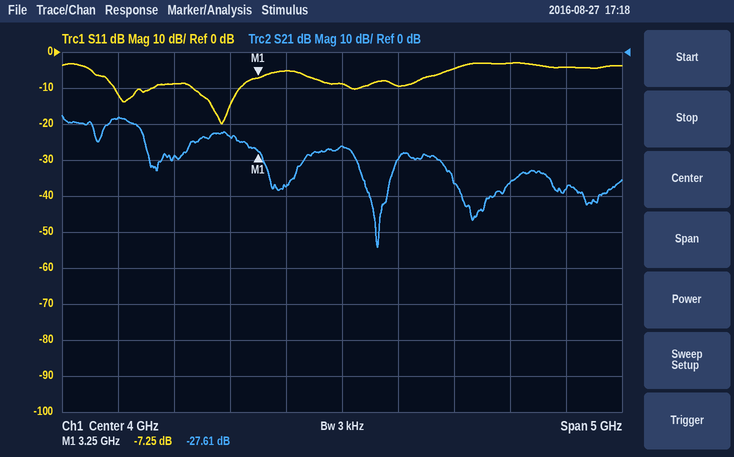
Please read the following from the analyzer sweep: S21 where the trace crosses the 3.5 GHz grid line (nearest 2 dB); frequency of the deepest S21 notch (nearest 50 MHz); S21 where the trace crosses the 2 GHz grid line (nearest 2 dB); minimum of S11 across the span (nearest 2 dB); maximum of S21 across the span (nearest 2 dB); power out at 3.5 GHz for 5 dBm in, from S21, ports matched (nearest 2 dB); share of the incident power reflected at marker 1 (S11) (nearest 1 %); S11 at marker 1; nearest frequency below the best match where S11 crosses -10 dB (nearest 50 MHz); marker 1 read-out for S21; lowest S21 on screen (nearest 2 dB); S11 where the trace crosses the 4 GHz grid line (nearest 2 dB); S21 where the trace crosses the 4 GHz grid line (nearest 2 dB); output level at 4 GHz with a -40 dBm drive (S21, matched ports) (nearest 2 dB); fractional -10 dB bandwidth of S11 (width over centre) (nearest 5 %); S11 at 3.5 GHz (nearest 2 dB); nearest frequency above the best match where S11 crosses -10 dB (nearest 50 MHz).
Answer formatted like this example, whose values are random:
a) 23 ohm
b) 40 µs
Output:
a) -38 dB
b) 4.30 GHz
c) -18 dB
d) -20 dB
e) -18 dB
f) -32 dBm
g) 19 %
h) -7.25 dB
i) 2.65 GHz
j) -27.61 dB
k) -54 dB
l) -8 dB
m) -26 dB
n) -66 dBm
o) 15 %
p) -6 dB
q) 3.10 GHz
